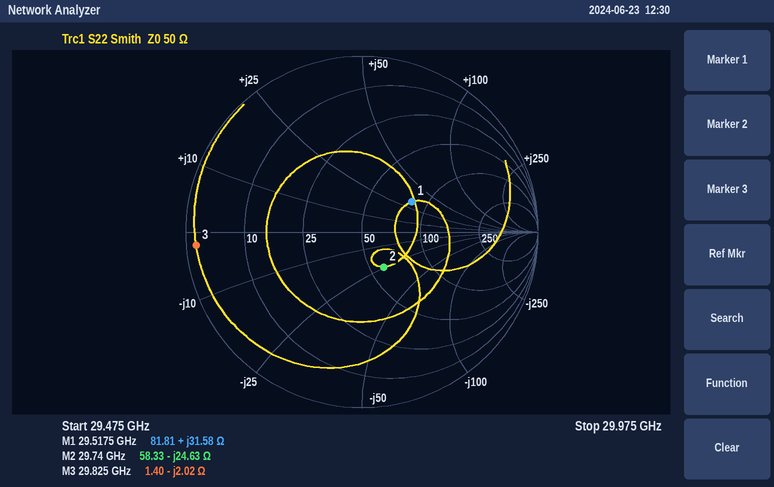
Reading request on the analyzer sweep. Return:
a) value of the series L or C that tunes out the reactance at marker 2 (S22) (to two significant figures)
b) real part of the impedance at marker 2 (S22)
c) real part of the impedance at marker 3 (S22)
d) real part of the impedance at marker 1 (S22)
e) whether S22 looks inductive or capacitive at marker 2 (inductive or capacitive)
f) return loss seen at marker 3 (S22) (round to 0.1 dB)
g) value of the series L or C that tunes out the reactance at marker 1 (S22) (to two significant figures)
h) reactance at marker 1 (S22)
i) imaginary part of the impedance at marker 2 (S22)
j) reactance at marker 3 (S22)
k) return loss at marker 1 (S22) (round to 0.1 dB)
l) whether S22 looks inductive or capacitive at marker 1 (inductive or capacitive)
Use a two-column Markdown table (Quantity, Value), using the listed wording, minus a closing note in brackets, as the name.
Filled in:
| Quantity | Value |
|---|---|
| value of the series L or C that tunes out the reactance at marker 2 (S22) | 130 pH |
| real part of the impedance at marker 2 | 58.33 Ω |
| real part of the impedance at marker 3 | 1.40 Ω |
| real part of the impedance at marker 1 | 81.81 Ω |
| whether S22 looks inductive or capacitive at marker 2 | capacitive |
| return loss seen at marker 3 (S22) | 0.5 dB |
| value of the series L or C that tunes out the reactance at marker 1 (S22) | 170 fF |
| reactance at marker 1 | +31.58 Ω |
| imaginary part of the impedance at marker 2 | -24.63 Ω |
| reactance at marker 3 | -2.02 Ω |
| return loss at marker 1 (S22) | 9.6 dB |
| whether S22 looks inductive or capacitive at marker 1 | inductive |
